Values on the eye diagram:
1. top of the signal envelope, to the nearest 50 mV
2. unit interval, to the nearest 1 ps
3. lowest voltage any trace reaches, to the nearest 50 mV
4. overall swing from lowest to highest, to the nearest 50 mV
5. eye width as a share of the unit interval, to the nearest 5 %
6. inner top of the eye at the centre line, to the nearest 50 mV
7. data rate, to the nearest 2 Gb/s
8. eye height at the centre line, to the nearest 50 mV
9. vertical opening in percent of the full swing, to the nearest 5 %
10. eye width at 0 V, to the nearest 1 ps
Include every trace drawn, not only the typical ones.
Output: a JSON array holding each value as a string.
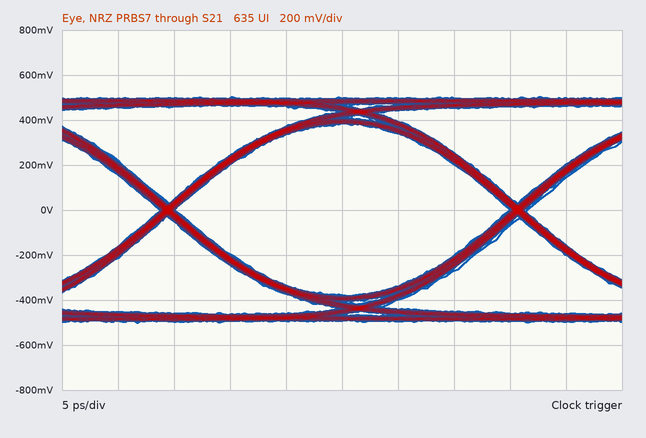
["500 mV", "31 ps", "-500 mV", "1.00 V", "95 %", "400 mV", "32 Gb/s", "750 mV", "75 %", "30 ps"]
